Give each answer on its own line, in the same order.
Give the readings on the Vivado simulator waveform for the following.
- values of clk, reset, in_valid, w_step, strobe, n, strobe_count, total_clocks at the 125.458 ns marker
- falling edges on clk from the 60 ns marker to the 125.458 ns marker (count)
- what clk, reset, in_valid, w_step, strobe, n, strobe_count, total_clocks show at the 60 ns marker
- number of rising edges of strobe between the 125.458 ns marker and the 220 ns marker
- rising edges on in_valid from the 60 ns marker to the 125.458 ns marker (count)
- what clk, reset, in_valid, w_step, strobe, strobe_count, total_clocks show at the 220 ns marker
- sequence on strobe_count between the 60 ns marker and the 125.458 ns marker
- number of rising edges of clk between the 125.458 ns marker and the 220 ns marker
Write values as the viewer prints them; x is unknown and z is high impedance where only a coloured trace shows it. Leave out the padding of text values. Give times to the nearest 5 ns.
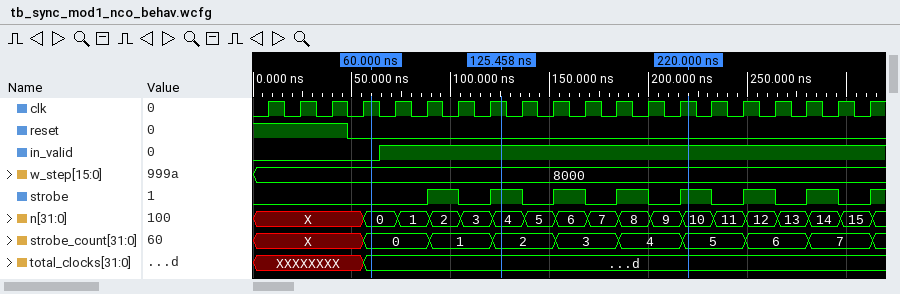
clk=1, reset=0, in_valid=1, w_step=8000, strobe=1, n=4, strobe_count=2, total_clocks=d
4
clk=1, reset=0, in_valid=0, w_step=8000, strobe=0, n=0, strobe_count=0, total_clocks=d
3
1
clk=1, reset=0, in_valid=1, w_step=8000, strobe=1, strobe_count=5, total_clocks=d
0, 1, 2
6
